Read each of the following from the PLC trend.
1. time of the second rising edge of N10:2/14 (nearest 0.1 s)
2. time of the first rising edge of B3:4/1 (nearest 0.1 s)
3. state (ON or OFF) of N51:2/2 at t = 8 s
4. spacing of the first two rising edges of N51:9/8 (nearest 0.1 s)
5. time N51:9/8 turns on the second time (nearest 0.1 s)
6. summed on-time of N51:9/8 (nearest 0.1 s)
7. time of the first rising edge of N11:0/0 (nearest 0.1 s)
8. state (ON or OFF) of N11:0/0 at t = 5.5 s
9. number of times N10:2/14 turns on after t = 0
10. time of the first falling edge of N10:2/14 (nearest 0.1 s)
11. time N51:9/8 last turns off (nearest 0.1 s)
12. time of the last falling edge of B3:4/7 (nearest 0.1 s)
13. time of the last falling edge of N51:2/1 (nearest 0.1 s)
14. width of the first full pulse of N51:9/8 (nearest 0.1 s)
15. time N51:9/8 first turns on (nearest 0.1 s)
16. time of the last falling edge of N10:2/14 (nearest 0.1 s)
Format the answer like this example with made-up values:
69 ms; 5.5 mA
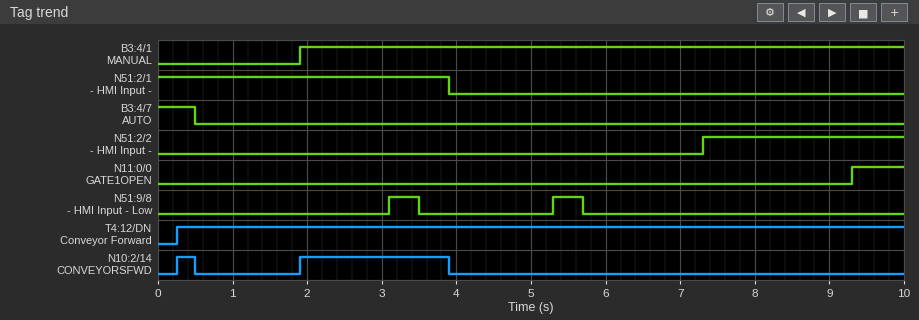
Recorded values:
1.9 s; 1.9 s; ON; 2.2 s; 5.3 s; 0.8 s; 9.3 s; OFF; 2; 0.5 s; 5.7 s; 0.5 s; 3.9 s; 0.4 s; 3.1 s; 3.9 s
